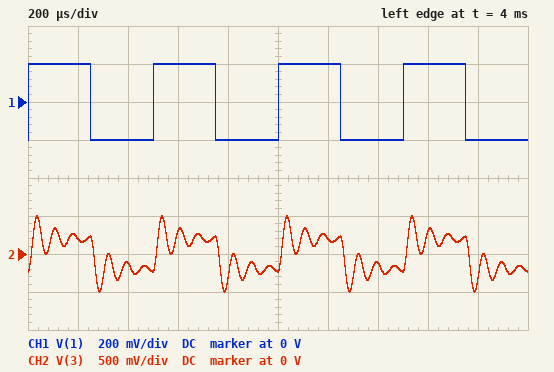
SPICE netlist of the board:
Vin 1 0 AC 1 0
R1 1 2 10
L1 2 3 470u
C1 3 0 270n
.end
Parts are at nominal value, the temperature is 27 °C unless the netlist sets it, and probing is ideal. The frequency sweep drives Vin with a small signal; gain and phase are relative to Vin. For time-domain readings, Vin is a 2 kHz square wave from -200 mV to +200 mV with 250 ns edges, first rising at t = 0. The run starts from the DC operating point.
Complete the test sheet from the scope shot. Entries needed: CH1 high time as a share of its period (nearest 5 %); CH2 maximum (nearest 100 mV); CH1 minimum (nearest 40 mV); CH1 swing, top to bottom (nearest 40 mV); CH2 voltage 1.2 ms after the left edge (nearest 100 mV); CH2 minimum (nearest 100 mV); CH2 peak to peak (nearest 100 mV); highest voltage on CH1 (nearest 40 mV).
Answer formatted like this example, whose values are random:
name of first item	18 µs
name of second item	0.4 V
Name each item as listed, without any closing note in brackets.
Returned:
CH1 high time as a share of its period	50 %
CH2 maximum	500 mV
CH1 minimum	-200 mV
CH1 swing, top to bottom	400 mV
CH2 voltage 1.2 ms after the left edge	200 mV
CH2 minimum	-500 mV
CH2 peak to peak	1.0 V
highest voltage on CH1	200 mV
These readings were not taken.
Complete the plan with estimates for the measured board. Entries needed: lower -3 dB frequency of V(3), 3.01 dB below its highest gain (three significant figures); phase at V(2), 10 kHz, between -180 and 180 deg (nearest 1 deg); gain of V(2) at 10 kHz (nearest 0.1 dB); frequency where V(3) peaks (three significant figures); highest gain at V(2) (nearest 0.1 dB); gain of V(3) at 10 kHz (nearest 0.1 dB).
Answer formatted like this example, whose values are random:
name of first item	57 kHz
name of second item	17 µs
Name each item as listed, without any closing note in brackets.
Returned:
lower -3 dB frequency of V(3), 3.01 dB below its highest gain	12.1 kHz
phase at V(2), 10 kHz, between -180 and 180 deg	-19 deg
gain of V(2) at 10 kHz	-0.5 dB
frequency where V(3) peaks	13.9 kHz
highest gain at V(2)	0 dB
gain of V(3) at 10 kHz	5.6 dB
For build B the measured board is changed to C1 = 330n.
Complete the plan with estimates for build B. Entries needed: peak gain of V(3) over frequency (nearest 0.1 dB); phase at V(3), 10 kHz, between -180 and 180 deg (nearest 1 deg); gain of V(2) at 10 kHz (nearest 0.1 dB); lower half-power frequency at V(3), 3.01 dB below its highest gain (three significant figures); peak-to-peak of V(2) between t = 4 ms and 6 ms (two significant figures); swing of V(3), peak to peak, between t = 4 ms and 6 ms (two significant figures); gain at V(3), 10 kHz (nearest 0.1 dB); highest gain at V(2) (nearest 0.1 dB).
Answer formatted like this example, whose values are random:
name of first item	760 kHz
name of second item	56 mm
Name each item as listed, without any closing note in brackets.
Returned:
peak gain of V(3) over frequency	11.6 dB
phase at V(3), 10 kHz, between -180 and 180 deg	-28 deg
gain of V(2) at 10 kHz	-1.1 dB
lower half-power frequency at V(3), 3.01 dB below its highest gain	10.7 kHz
peak-to-peak of V(2) between t = 4 ms and 6 ms	510 mV
swing of V(3), peak to peak, between t = 4 ms and 6 ms	900 mV
gain at V(3), 10 kHz	7.1 dB
highest gain at V(2)	0 dB
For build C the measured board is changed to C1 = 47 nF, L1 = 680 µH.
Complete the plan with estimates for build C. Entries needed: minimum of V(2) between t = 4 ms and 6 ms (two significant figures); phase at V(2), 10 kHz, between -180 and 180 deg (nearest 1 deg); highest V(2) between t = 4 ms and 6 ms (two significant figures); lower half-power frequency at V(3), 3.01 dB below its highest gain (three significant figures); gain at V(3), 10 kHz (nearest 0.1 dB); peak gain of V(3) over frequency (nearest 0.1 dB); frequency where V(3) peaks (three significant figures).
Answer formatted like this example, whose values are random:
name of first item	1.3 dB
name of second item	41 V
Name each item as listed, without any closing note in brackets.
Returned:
minimum of V(2) between t = 4 ms and 6 ms	-220 mV
phase at V(2), 10 kHz, between -180 and 180 deg	-2 deg
highest V(2) between t = 4 ms and 6 ms	220 mV
lower half-power frequency at V(3), 3.01 dB below its highest gain	26.9 kHz
gain at V(3), 10 kHz	1.2 dB
peak gain of V(3) over frequency	21.6 dB
frequency where V(3) peaks	28.1 kHz
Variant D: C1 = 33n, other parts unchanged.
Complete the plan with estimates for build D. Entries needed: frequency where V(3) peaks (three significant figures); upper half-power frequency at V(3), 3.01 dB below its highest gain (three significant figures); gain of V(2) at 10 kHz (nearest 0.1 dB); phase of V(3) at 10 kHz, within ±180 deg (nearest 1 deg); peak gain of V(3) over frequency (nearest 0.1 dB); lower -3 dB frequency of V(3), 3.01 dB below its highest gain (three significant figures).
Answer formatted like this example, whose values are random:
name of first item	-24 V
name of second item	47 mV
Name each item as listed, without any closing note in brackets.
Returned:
frequency where V(3) peaks	40.3 kHz
upper half-power frequency at V(3), 3.01 dB below its highest gain	42.0 kHz
gain of V(2) at 10 kHz	0 dB
phase of V(3) at 10 kHz, within ±180 deg	-1 deg
peak gain of V(3) over frequency	21.5 dB
lower -3 dB frequency of V(3), 3.01 dB below its highest gain	38.6 kHz
